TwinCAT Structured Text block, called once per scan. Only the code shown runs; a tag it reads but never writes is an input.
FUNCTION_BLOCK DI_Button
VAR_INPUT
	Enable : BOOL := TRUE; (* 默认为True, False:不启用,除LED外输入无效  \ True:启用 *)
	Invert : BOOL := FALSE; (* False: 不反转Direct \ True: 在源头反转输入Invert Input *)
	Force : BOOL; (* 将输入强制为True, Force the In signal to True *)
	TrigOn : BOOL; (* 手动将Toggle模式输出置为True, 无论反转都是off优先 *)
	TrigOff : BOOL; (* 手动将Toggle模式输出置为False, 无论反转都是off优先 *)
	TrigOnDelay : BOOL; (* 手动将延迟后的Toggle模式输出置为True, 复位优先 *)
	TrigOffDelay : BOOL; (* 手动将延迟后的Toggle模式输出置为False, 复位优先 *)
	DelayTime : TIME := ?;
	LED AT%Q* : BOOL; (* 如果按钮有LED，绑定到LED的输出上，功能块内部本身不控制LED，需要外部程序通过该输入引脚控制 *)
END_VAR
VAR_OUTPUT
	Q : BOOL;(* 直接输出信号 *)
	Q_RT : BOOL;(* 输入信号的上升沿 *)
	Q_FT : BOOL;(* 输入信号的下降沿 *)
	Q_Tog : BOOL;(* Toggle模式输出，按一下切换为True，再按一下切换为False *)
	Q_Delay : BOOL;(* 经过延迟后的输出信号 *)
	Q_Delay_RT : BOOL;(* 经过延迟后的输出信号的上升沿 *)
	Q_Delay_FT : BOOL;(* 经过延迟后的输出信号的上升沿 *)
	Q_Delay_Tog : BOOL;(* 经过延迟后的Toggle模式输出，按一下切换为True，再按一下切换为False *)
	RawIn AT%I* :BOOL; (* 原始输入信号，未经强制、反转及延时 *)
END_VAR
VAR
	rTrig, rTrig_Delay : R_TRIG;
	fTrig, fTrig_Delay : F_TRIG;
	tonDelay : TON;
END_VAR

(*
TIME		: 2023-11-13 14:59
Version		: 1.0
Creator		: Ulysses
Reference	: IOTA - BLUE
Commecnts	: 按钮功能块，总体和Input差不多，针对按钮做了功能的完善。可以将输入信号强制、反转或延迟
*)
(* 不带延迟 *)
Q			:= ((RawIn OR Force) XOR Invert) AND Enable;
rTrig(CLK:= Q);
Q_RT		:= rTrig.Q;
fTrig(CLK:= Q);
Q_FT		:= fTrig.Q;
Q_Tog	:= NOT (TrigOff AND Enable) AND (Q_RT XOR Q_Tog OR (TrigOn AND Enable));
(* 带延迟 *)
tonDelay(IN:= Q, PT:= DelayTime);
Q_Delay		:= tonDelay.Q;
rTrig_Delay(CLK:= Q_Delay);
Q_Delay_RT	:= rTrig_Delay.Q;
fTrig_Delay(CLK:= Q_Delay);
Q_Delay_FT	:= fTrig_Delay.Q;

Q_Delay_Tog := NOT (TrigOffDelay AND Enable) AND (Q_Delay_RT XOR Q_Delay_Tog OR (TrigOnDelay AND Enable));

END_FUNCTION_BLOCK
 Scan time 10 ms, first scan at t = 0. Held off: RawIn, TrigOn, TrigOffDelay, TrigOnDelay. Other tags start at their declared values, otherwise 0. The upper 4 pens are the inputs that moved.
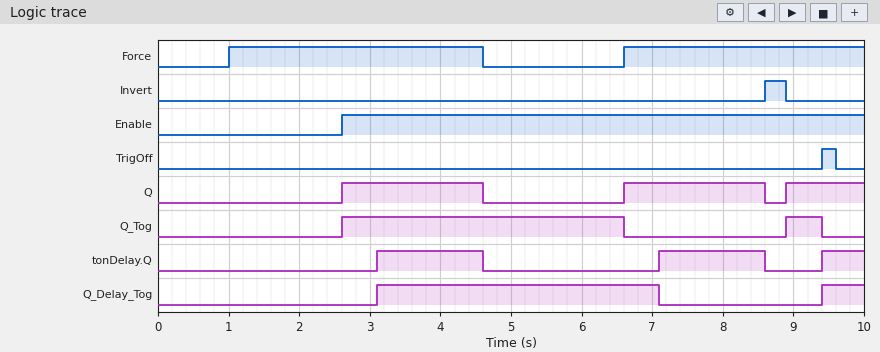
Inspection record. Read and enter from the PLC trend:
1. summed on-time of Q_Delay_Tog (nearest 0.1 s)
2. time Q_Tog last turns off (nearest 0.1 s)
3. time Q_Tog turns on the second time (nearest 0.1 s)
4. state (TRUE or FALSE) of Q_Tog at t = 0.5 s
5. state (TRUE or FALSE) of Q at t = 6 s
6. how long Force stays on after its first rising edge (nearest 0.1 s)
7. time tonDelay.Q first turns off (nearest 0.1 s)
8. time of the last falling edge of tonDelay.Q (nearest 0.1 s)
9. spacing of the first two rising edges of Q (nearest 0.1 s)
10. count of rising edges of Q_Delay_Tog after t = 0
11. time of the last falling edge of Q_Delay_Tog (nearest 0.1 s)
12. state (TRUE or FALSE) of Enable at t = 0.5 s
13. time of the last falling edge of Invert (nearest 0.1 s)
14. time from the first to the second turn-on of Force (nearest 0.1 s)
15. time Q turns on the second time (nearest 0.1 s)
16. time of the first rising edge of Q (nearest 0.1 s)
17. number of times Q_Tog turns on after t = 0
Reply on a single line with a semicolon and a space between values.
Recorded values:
4.6 s; 9.4 s; 8.9 s; FALSE; FALSE; 3.6 s; 4.6 s; 8.6 s; 4.0 s; 2; 7.1 s; FALSE; 8.9 s; 5.6 s; 6.6 s; 2.6 s; 2
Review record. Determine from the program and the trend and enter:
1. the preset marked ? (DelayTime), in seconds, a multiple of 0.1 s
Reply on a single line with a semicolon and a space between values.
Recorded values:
0.5 s
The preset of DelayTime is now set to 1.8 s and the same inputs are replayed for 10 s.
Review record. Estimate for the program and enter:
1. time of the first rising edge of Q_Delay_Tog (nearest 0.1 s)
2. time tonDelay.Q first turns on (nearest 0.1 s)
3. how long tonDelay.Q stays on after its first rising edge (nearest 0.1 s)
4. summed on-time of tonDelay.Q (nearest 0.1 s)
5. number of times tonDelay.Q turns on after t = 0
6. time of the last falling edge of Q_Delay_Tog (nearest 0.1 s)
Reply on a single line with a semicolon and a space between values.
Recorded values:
4.4 s; 4.4 s; 0.2 s; 0.4 s; 2; 8.4 s
